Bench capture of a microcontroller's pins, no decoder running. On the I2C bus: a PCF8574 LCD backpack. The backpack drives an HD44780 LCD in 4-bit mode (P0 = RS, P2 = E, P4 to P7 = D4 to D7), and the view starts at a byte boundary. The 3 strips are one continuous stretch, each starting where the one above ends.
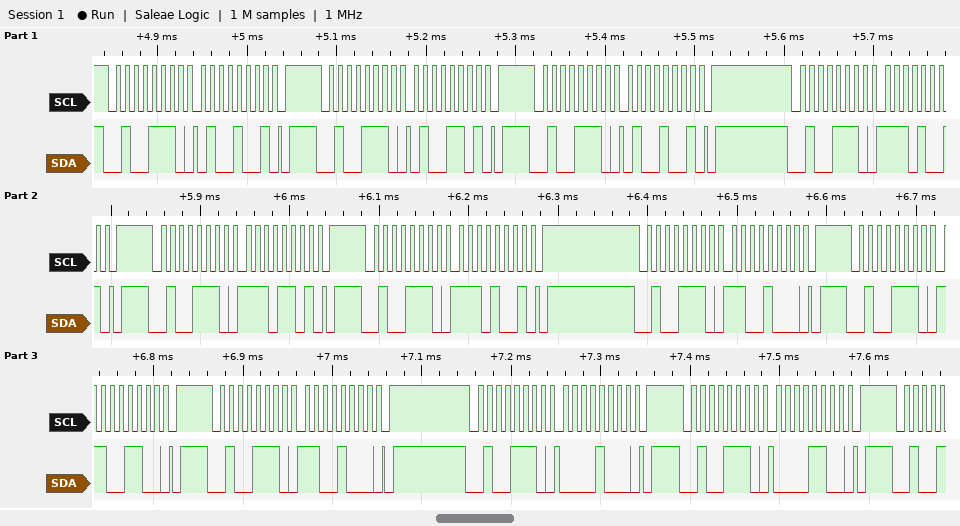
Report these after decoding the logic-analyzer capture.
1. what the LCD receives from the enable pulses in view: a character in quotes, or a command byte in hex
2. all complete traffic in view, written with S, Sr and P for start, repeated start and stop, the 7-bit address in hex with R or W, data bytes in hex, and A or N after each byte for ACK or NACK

'N'
S 27W A 49 A P S 27W A 4D A P S 27W A 49 A P S 27W A E9 A P S 27W A ED A P S 27W A E9 A P S 27W A C8 A P S 27W A CC A P S 27W A C8 A P S 27W A 08 A P S 27W A 0C A P
